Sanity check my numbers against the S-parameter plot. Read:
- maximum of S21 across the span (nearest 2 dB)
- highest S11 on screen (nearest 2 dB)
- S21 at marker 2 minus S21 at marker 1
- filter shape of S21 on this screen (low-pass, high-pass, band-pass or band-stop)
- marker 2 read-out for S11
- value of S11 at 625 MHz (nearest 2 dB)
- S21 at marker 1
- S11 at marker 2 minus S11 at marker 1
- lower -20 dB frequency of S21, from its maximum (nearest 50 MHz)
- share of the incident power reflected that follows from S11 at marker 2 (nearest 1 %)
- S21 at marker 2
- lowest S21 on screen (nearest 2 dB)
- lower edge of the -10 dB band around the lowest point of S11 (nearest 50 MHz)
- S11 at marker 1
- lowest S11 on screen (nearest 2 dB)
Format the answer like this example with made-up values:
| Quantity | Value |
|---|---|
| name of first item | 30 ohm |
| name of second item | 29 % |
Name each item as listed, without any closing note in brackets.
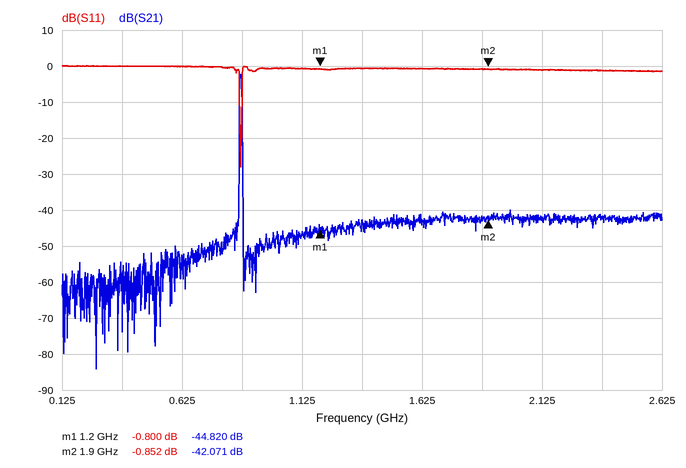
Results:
| Quantity | Value |
|---|---|
| maximum of S21 across the span | -2 dB |
| highest S11 on screen | 0 dB |
| S21 at marker 2 minus S21 at marker 1 | 2.749 dB |
| filter shape of S21 on this screen | band-pass |
| marker 2 read-out for S11 | -0.852 dB |
| value of S11 at 625 MHz | 0 dB |
| S21 at marker 1 | -44.820 dB |
| S11 at marker 2 minus S11 at marker 1 | -0.052 dB |
| lower -20 dB frequency of S21, from its maximum | 850 MHz |
| share of the incident power reflected that follows from S11 at marker 2 | 82 % |
| S21 at marker 2 | -42.071 dB |
| lowest S21 on screen | -84 dB |
| lower edge of the -10 dB band around the lowest point of S11 | 850 MHz |
| S11 at marker 1 | -0.800 dB |
| lowest S11 on screen | -28 dB |
